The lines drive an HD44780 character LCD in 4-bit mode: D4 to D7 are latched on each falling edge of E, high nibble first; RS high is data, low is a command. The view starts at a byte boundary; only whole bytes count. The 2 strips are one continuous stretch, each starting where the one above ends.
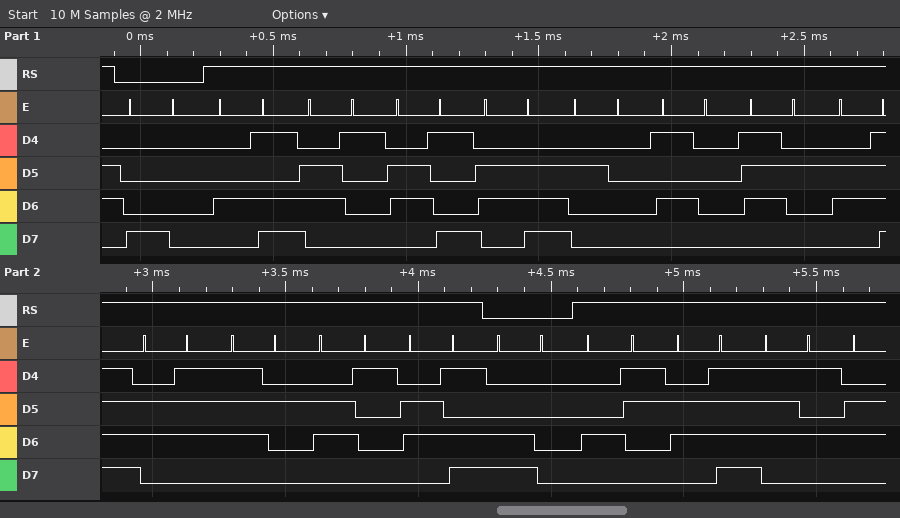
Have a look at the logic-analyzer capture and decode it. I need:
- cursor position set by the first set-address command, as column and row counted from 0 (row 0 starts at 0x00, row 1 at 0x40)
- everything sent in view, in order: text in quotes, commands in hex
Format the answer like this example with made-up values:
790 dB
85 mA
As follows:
column 0, row 0
0x80 "Main Program" 0xC0 "Cou"
